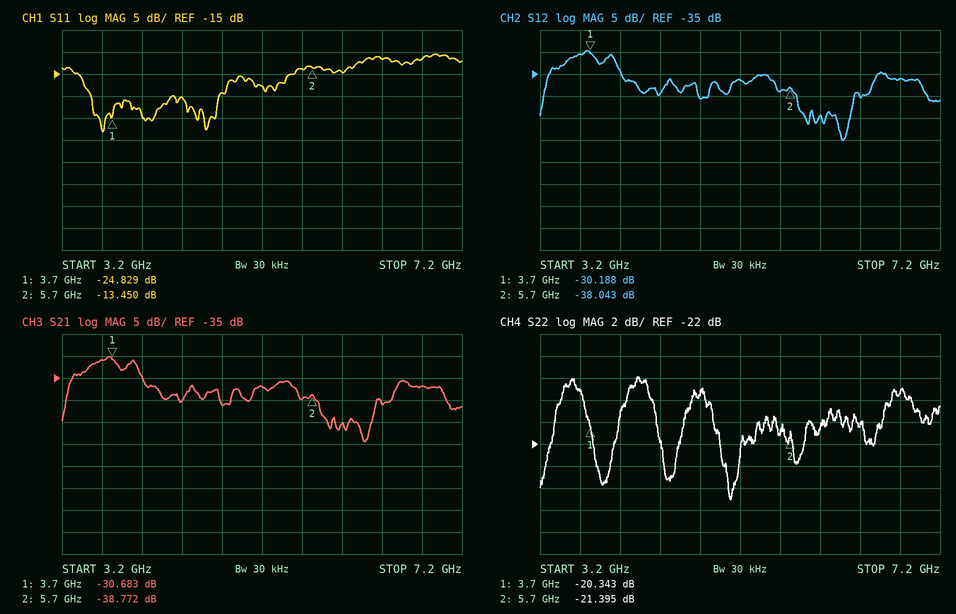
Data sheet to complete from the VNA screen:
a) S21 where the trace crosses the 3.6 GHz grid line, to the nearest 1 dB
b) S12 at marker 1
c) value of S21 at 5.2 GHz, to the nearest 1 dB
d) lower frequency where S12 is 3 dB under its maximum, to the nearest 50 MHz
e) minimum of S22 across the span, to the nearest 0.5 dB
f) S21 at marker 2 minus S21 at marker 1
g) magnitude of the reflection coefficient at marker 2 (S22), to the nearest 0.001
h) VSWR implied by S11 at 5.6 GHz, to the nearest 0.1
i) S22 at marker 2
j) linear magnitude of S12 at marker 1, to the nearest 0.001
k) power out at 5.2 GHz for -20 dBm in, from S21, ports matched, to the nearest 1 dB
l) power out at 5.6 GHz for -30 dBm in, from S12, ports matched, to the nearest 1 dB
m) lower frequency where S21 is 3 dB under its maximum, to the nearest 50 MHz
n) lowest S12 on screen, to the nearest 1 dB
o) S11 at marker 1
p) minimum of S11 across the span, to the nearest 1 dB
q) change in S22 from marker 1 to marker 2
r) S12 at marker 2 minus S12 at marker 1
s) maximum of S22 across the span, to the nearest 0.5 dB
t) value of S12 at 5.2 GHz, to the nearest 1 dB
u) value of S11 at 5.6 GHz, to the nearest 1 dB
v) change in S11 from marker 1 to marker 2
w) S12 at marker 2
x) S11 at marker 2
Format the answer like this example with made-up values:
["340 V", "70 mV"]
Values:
["-31 dB", "-30.188 dB", "-37 dB", "3.45 GHz", "-27.0 dB", "-8.089 dB", "0.085", "1.5", "-21.395 dB", "0.031", "-57 dBm", "-69 dBm", "3.45 GHz", "-50 dB", "-24.829 dB", "-28 dB", "-1.052 dB", "-7.855 dB", "-16.0 dB", "-36 dB", "-14 dB", "11.379 dB", "-38.043 dB", "-13.450 dB"]
